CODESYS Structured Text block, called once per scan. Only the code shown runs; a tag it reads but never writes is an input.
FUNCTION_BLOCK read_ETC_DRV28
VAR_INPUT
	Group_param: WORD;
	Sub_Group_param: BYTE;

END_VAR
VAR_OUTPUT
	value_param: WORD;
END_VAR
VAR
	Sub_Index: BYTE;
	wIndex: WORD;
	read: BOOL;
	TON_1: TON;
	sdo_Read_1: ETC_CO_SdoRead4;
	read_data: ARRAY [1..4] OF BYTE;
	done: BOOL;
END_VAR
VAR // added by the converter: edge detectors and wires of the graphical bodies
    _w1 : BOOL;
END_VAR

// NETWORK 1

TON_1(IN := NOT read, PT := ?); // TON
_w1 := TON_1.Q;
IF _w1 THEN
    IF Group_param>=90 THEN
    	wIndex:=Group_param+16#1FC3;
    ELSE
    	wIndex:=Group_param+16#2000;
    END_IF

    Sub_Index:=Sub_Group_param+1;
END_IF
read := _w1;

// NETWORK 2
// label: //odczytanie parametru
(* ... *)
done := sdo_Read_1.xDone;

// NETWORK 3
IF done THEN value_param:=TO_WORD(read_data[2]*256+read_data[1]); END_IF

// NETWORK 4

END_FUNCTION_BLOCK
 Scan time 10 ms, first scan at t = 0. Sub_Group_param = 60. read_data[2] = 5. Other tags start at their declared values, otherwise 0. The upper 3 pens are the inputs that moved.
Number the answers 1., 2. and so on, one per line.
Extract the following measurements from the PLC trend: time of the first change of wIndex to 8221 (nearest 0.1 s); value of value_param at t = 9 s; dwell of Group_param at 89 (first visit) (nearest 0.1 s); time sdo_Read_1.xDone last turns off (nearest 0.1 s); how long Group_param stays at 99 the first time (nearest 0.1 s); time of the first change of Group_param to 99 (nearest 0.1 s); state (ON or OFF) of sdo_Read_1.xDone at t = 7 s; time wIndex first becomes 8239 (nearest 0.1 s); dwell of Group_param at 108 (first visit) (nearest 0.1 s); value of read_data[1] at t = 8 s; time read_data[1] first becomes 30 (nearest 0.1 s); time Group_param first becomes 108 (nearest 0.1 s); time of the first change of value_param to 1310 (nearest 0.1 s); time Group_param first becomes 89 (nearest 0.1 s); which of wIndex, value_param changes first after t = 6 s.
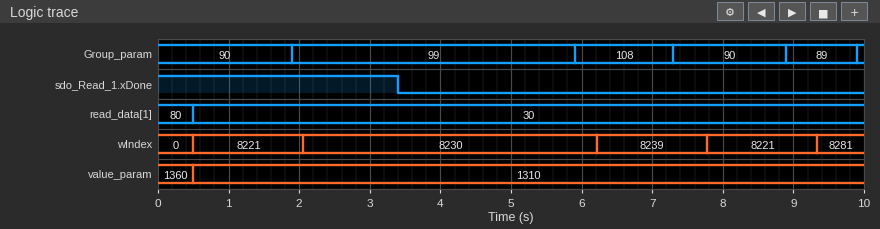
1. 0.5 s
2. 1310
3. 1.0 s
4. 3.4 s
5. 4.0 s
6. 1.9 s
7. OFF
8. 6.2 s
9. 1.4 s
10. 30
11. 0.5 s
12. 5.9 s
13. 0.5 s
14. 8.9 s
15. wIndex
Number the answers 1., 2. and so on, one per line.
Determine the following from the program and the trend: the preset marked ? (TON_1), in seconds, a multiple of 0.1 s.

1. 0.5 s
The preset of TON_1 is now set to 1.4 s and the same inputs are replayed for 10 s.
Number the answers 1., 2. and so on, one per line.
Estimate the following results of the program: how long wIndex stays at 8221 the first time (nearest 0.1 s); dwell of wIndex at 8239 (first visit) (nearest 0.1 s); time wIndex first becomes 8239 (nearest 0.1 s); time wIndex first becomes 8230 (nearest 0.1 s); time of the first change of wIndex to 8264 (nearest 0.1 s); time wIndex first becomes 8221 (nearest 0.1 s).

1. 1.4 s
2. 1.4 s
3. 7.1 s
4. 2.8 s
5. 9.9 s
6. 1.4 s
